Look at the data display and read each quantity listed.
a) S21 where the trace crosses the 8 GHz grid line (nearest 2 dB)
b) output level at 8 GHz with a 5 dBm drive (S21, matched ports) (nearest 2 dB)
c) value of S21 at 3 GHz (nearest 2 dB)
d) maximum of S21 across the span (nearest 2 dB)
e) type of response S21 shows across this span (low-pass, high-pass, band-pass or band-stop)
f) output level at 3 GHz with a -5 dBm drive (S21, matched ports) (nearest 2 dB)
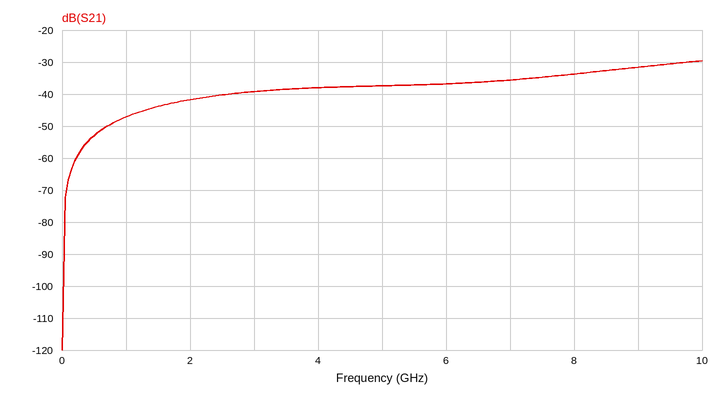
-34 dB
-28 dBm
-40 dB
-30 dB
high-pass
-44 dBm
